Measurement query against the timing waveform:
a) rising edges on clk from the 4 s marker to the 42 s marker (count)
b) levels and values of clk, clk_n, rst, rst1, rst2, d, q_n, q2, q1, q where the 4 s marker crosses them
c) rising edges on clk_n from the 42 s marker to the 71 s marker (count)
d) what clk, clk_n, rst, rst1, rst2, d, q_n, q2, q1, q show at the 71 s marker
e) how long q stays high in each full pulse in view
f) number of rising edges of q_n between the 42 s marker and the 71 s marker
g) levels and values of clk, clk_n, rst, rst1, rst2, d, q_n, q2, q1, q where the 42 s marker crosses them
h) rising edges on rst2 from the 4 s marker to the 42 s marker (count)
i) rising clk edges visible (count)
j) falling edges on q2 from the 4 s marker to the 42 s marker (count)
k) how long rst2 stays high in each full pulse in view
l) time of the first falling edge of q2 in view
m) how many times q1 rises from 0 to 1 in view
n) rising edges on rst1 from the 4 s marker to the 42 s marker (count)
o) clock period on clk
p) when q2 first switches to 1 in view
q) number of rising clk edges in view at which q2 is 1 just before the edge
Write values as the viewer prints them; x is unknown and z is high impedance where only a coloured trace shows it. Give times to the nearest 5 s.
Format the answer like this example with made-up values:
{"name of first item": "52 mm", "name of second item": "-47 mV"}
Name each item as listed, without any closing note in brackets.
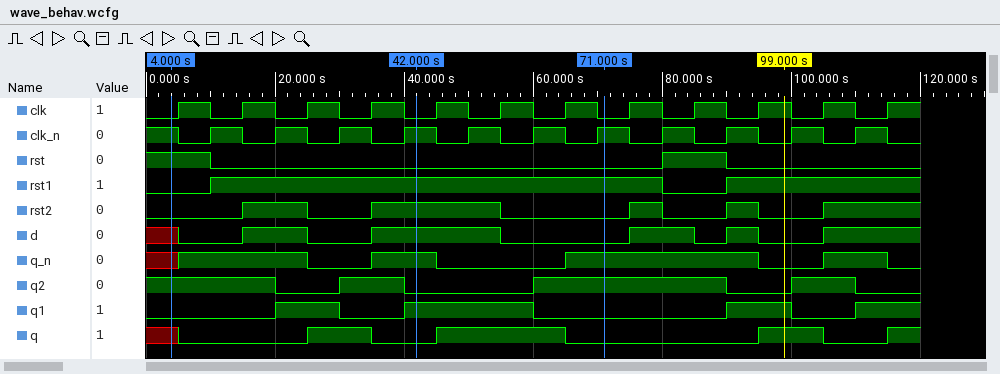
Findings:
{"rising edges on clk from the 4 s marker to the 42 s marker": "4", "levels and values of clk, clk_n, rst, rst1, rst2, d, q_n, q2, q1, q where the 4 s marker crosses them": "clk=0, clk_n=1, rst=1, rst1=0, rst2=0, d=x, q_n=x, q2=1, q1=0, q=x", "rising edges on clk_n from the 42 s marker to the 71 s marker": "3", "what clk, clk_n, rst, rst1, rst2, d, q_n, q2, q1, q show at the 71 s marker": "clk=0, clk_n=1, rst=0, rst1=1, rst2=0, d=0, q_n=1, q2=1, q1=0, q=0", "how long q stays high in each full pulse in view": "10 s, 20 s, 10 s", "number of rising edges of q_n between the 42 s marker and the 71 s marker": "1", "levels and values of clk, clk_n, rst, rst1, rst2, d, q_n, q2, q1, q where the 42 s marker crosses them": "clk=0, clk_n=1, rst=0, rst1=1, rst2=1, d=1, q_n=1, q2=0, q1=1, q=0", "rising edges on rst2 from the 4 s marker to the 42 s marker": "2", "rising clk edges visible": "12", "falling edges on q2 from the 4 s marker to the 42 s marker": "2", "how long rst2 stays high in each full pulse in view": "10 s, 20 s, 5 s, 5 s", "time of the first falling edge of q2 in view": "20 s", "how many times q1 rises from 0 to 1 in view": "4", "rising edges on rst1 from the 4 s marker to the 42 s marker": "1", "clock period on clk": "10 s", "when q2 first switches to 1 in view": "30 s", "number of rising clk edges in view at which q2 is 1 just before the edge": "7"}
